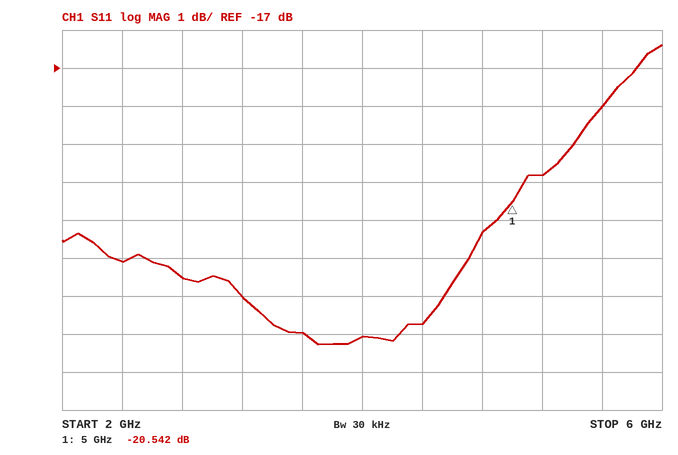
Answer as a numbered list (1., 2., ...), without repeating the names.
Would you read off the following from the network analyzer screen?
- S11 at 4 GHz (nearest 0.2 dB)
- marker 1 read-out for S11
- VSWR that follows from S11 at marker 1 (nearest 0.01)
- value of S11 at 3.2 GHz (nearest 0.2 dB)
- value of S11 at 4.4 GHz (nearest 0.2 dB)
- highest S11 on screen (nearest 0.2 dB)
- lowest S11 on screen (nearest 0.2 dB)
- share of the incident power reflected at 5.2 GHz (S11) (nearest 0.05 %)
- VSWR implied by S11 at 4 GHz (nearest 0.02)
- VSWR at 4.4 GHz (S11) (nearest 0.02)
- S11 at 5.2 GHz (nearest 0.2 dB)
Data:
1. -24.0 dB
2. -20.542 dB
3. 1.21
4. -23.0 dB
5. -23.8 dB
6. -16.4 dB
7. -24.2 dB
8. 1.05 %
9. 1.14
10. 1.14
11. -19.8 dB
